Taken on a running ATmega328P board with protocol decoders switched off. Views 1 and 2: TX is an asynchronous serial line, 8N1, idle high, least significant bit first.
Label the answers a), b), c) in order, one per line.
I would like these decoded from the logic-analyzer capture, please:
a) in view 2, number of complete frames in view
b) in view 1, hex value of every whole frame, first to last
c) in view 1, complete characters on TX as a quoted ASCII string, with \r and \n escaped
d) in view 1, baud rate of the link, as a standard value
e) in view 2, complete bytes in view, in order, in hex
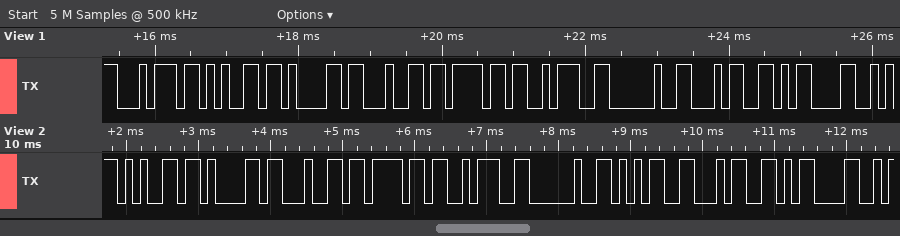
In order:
a) 9
b) 0x74 0x65 0x61 0x64 0x6F 0x3A 0x20 0x34 0x0D
c) "teado: 4\r"
d) 9600 baud
e) 0x65 0x61 0x64 0x6F 0x3A 0x20 0x35 0x34 0x0D
